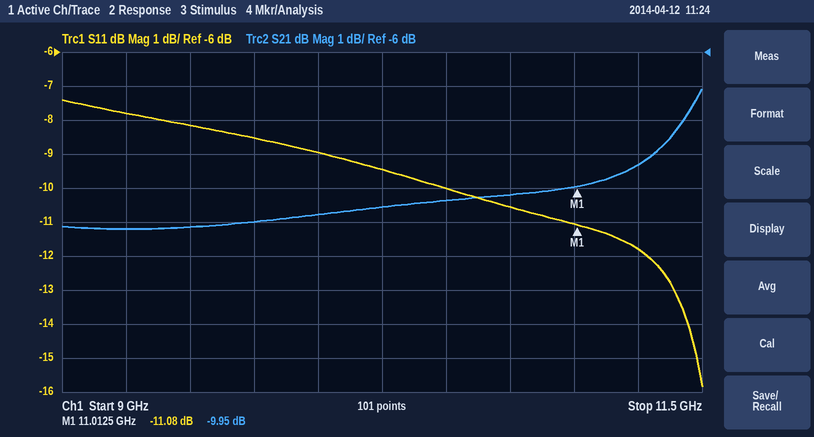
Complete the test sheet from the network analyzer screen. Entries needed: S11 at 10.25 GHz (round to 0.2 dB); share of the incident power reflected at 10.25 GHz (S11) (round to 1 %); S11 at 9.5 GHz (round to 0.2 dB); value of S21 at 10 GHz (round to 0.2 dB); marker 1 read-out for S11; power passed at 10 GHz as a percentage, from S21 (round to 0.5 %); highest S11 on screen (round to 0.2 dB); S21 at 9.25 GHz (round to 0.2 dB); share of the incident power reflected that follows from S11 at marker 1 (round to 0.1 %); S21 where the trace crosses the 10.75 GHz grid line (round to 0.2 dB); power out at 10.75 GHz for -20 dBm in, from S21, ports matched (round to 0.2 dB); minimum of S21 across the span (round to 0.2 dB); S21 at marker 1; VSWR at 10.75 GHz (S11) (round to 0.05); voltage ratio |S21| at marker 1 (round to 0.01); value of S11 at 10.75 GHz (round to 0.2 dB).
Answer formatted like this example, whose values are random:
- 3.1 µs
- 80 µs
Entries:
- -9.4 dB
- 11 %
- -8.2 dB
- -10.8 dB
- -11.08 dB
- 8.5 %
- -7.4 dB
- -11.2 dB
- 7.8 %
- -10.2 dB
- -30.2 dBm
- -11.2 dB
- -9.95 dB
- 1.85
- 0.32
- -10.6 dB
